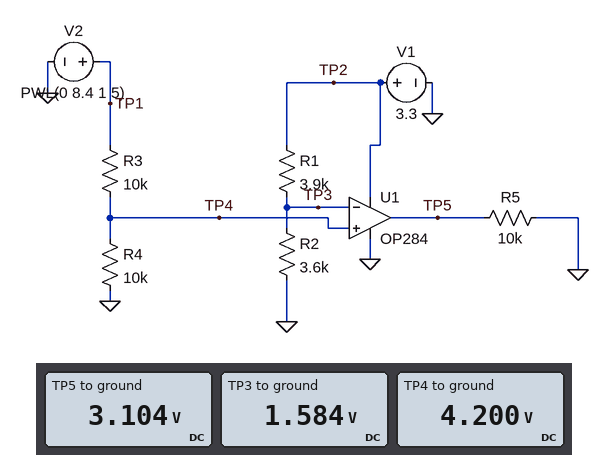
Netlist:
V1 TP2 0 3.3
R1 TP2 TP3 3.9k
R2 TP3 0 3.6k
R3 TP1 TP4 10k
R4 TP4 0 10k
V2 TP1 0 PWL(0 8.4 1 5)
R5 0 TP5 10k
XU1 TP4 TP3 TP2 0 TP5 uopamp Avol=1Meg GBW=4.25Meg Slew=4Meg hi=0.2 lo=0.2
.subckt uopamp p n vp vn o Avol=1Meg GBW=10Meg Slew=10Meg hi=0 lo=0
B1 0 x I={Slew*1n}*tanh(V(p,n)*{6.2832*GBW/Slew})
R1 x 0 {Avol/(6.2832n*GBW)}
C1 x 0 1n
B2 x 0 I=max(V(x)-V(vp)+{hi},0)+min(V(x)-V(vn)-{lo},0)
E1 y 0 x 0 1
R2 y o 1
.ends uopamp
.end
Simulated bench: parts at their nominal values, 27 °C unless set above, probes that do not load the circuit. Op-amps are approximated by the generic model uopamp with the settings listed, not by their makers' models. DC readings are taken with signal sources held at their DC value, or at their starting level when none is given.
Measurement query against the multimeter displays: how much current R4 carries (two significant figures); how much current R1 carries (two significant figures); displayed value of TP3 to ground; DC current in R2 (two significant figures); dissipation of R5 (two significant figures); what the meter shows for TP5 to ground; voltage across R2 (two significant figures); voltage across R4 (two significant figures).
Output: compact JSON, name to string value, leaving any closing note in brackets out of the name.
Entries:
{"how much current R4 carries": "420 µA", "how much current R1 carries": "440 µA", "displayed value of TP3 to ground": "1.584 V", "DC current in R2": "440 µA", "dissipation of R5": "960 µW", "what the meter shows for TP5 to ground": "3.104 V", "voltage across R2": "1.6 V", "voltage across R4": "4.2 V"}
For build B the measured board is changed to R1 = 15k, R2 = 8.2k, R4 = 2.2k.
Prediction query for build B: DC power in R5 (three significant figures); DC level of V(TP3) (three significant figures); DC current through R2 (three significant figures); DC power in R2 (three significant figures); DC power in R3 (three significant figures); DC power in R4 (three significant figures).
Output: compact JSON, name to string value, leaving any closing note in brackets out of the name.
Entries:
{"DC power in R5": "963 µW", "DC level of V(TP3)": "1.17 V", "DC current through R2": "142 µA", "DC power in R2": "166 µW", "DC power in R3": "4.74 mW", "DC power in R4": "1.04 mW"}
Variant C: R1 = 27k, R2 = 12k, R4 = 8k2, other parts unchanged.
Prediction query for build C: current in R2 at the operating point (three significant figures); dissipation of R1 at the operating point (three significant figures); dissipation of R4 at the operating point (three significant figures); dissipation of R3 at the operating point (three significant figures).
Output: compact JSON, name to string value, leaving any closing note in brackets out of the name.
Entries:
{"current in R2 at the operating point": "84.6 µA", "dissipation of R1 at the operating point": "193 µW", "dissipation of R4 at the operating point": "1.75 mW", "dissipation of R3 at the operating point": "2.13 mW"}
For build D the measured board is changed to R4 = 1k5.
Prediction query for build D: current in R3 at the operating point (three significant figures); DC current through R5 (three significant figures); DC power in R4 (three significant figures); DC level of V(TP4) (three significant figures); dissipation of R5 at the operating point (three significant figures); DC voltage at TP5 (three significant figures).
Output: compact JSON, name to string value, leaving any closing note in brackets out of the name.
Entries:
{"current in R3 at the operating point": "730 µA", "DC current through R5": "19.6 µA", "DC power in R4": "800 µW", "DC level of V(TP4)": "1.10 V", "dissipation of R5 at the operating point": "3.84 µW", "DC voltage at TP5": "196 mV"}
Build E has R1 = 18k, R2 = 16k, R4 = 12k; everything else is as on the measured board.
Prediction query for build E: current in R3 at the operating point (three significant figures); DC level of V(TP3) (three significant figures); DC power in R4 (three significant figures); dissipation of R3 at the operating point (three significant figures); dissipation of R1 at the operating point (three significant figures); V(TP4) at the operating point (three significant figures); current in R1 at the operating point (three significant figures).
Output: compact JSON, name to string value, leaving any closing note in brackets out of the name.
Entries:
{"current in R3 at the operating point": "382 µA", "DC level of V(TP3)": "1.55 V", "DC power in R4": "1.75 mW", "dissipation of R3 at the operating point": "1.46 mW", "dissipation of R1 at the operating point": "170 µW", "V(TP4) at the operating point": "4.58 V", "current in R1 at the operating point": "97.1 µA"}
